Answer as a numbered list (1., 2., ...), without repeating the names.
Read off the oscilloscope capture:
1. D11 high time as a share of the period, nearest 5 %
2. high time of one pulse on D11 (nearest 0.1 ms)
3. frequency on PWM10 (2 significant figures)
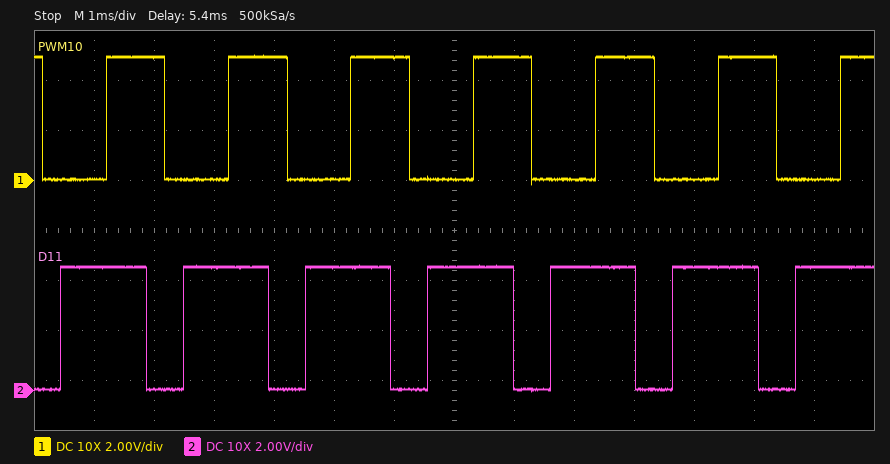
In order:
1. 70 %
2. 1.4 ms
3. 490 Hz
